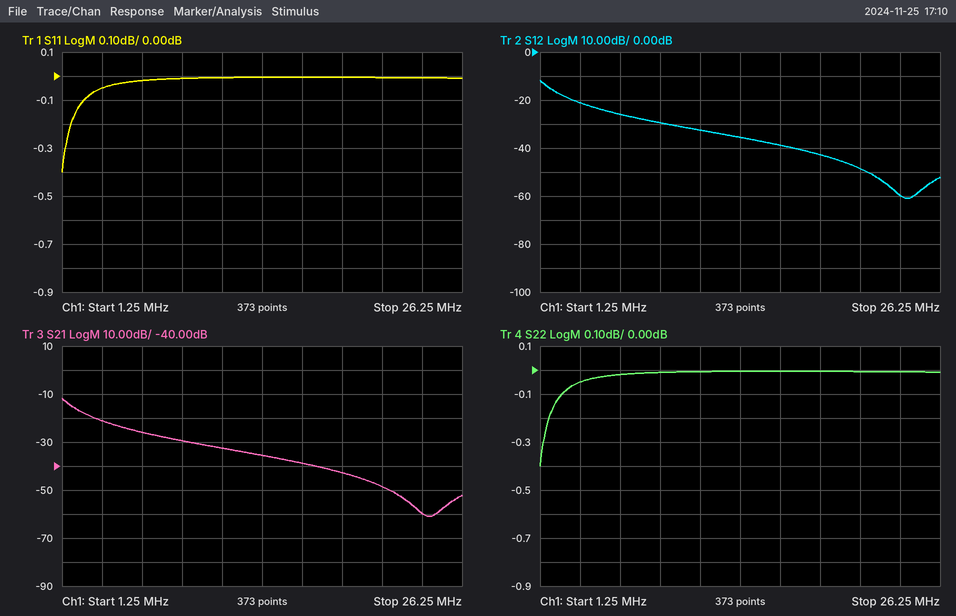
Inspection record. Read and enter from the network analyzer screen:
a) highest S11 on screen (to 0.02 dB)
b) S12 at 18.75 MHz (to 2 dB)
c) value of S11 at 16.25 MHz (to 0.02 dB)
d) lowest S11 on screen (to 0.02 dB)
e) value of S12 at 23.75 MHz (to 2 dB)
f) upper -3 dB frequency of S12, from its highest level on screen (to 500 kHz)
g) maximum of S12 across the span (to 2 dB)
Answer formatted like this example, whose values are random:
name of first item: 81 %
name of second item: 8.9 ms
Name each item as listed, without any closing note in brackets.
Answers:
highest S11 on screen: 0.00 dB
S12 at 18.75 MHz: -42 dB
value of S11 at 16.25 MHz: 0.00 dB
lowest S11 on screen: -0.40 dB
value of S12 at 23.75 MHz: -60 dB
upper -3 dB frequency of S12, from its highest level on screen: 2.0 MHz
maximum of S12 across the span: -12 dB
